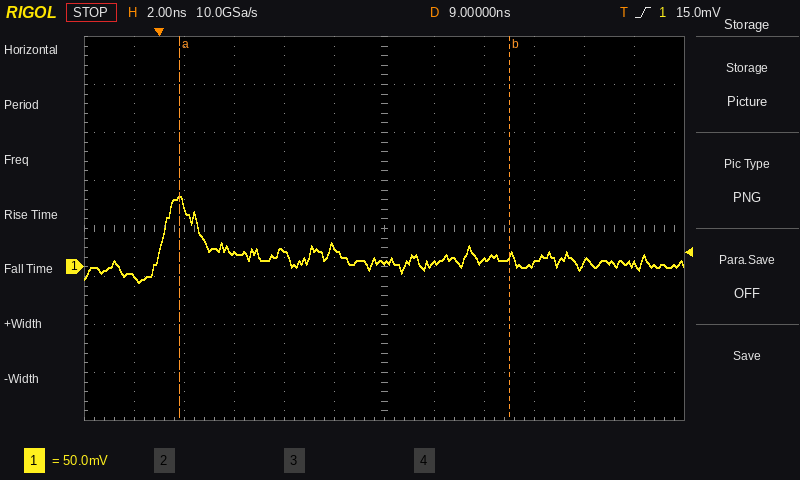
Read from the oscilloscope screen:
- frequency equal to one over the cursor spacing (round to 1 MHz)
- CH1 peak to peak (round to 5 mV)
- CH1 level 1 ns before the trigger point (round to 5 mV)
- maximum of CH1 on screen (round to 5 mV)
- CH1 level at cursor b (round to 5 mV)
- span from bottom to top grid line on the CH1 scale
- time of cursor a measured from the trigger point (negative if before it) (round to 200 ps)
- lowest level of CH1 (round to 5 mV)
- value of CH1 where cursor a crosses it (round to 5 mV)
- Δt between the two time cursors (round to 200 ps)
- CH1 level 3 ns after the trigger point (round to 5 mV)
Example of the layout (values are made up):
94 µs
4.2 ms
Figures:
76 MHz
90 mV
-10 mV
75 mV
10 mV
400 mV
+800 ps
-15 mV
70 mV
13.2 ns
15 mV
